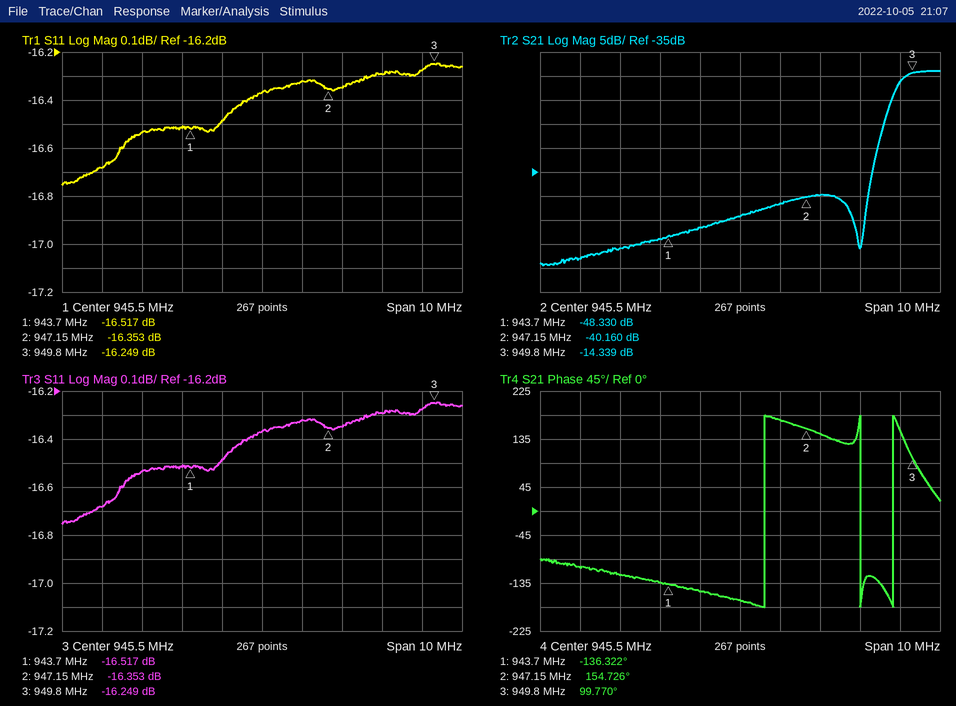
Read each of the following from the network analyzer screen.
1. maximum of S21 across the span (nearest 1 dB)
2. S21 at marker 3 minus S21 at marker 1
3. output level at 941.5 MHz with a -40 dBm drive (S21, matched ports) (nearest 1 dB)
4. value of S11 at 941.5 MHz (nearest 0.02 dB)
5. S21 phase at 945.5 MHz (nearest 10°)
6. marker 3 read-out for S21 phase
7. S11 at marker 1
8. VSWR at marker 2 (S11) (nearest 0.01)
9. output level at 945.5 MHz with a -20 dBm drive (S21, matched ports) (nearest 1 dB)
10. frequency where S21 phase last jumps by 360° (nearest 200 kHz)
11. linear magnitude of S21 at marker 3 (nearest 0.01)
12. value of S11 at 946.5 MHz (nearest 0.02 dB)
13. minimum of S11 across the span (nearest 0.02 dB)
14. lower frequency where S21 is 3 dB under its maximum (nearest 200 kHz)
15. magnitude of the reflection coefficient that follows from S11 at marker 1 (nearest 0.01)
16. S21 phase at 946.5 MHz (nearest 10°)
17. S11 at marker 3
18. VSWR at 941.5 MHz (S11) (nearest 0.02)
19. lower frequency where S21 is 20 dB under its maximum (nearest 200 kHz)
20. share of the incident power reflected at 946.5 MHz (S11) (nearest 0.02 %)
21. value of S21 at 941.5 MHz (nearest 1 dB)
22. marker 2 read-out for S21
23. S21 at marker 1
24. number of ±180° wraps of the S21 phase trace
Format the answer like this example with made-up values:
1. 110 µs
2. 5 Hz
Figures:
1. -14 dB
2. 33.991 dB
3. -93 dBm
4. -16.68 dB
5. -170°
6. 99.770°
7. -16.517 dB
8. 1.36
9. -64 dBm
10. 949.4 MHz
11. 0.19
12. -16.32 dB
13. -16.76 dB
14. 949.4 MHz
15. 0.15
16. 170°
17. -16.249 dB
18. 1.34
19. 948.8 MHz
20. 2.34 %
21. -53 dB
22. -40.160 dB
23. -48.330 dB
24. 3
